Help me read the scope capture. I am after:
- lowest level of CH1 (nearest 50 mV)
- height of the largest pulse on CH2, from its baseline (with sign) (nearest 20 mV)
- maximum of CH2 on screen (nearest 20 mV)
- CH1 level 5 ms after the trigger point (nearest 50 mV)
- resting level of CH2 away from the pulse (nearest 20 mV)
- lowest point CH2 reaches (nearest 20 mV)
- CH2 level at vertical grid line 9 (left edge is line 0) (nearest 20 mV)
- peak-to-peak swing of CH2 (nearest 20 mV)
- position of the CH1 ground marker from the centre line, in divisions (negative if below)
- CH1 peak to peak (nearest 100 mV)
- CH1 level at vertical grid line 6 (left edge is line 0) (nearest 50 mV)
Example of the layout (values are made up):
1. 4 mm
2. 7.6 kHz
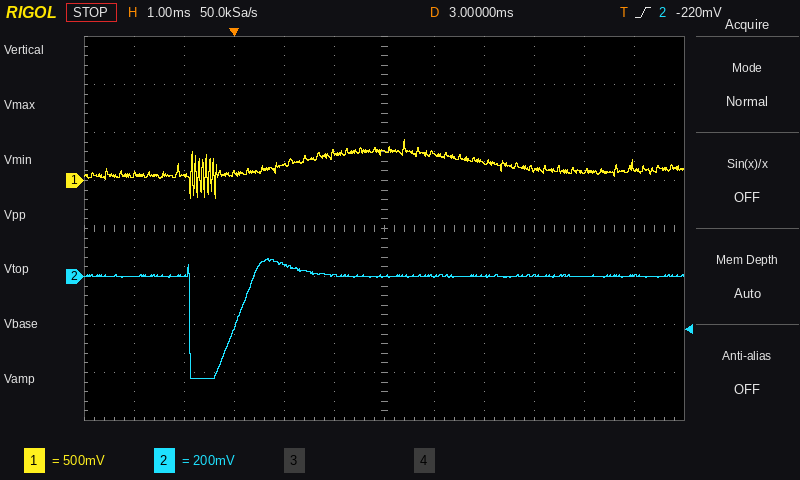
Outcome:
1. -200 mV
2. -420 mV
3. 80 mV
4. 200 mV
5. 0 mV
6. -420 mV
7. 0 mV
8. 500 mV
9. +1.0 div
10. 600 mV
11. 300 mV
